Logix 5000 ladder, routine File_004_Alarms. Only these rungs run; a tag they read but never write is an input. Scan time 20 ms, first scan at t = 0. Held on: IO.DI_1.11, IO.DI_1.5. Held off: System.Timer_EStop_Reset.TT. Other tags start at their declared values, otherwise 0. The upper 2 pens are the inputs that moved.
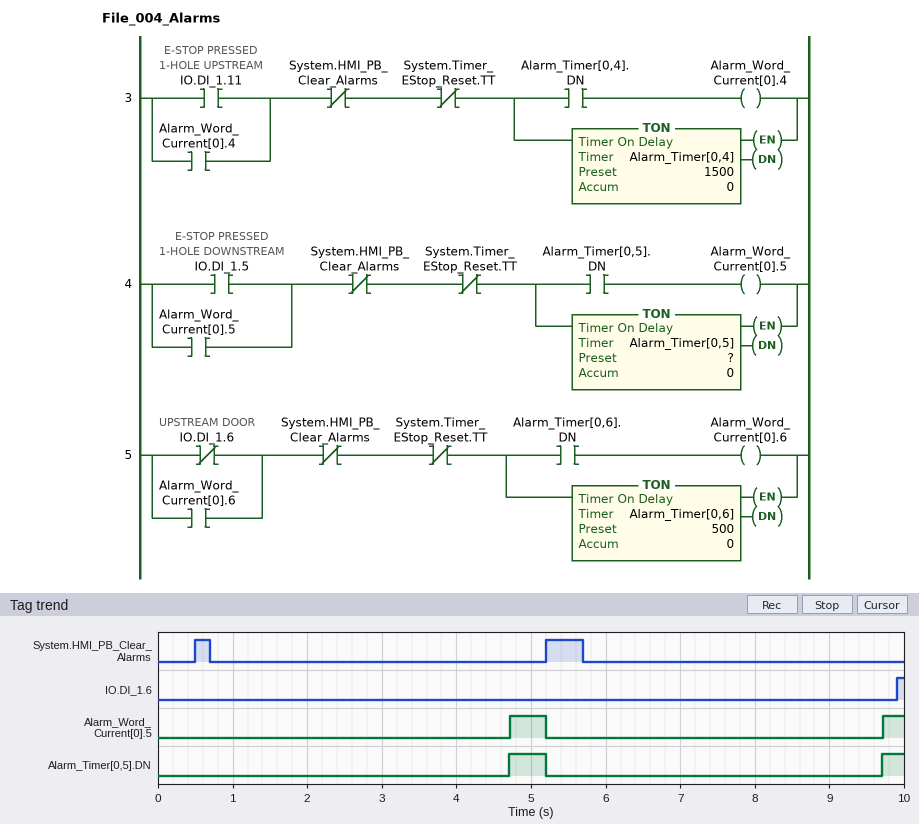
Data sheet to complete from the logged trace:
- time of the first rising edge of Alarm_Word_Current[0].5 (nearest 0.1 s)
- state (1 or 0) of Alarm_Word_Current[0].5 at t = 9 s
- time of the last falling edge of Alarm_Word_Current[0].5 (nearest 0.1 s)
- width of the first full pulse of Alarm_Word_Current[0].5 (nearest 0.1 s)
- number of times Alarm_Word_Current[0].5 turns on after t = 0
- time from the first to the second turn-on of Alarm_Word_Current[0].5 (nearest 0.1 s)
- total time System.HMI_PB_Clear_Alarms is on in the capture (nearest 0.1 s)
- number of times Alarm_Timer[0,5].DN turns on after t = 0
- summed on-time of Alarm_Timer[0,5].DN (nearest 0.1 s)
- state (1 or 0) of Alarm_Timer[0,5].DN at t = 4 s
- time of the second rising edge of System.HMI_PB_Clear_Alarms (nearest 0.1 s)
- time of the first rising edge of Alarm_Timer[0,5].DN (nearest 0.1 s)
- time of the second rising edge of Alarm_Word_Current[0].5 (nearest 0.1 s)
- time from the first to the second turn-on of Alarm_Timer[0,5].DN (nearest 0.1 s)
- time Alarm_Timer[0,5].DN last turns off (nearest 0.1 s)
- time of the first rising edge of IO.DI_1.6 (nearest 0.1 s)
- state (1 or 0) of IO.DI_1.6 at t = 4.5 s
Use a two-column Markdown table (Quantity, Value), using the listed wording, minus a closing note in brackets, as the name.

| Quantity | Value |
|---|---|
| time of the first rising edge of Alarm_Word_Current[0].5 | 4.7 s |
| state (1 or 0) of Alarm_Word_Current[0].5 at t = 9 s | 0 |
| time of the last falling edge of Alarm_Word_Current[0].5 | 5.2 s |
| width of the first full pulse of Alarm_Word_Current[0].5 | 0.5 s |
| number of times Alarm_Word_Current[0].5 turns on after t = 0 | 2 |
| time from the first to the second turn-on of Alarm_Word_Current[0].5 | 5.0 s |
| total time System.HMI_PB_Clear_Alarms is on in the capture | 0.7 s |
| number of times Alarm_Timer[0,5].DN turns on after t = 0 | 2 |
| summed on-time of Alarm_Timer[0,5].DN | 0.8 s |
| state (1 or 0) of Alarm_Timer[0,5].DN at t = 4 s | 0 |
| time of the second rising edge of System.HMI_PB_Clear_Alarms | 5.2 s |
| time of the first rising edge of Alarm_Timer[0,5].DN | 4.7 s |
| time of the second rising edge of Alarm_Word_Current[0].5 | 9.7 s |
| time from the first to the second turn-on of Alarm_Timer[0,5].DN | 5.0 s |
| time Alarm_Timer[0,5].DN last turns off | 5.2 s |
| time of the first rising edge of IO.DI_1.6 | 9.9 s |
| state (1 or 0) of IO.DI_1.6 at t = 4.5 s | 0 |
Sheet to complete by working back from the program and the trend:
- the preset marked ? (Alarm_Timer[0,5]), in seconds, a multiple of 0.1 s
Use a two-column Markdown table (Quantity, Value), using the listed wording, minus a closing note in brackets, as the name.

| Quantity | Value |
|---|---|
| the preset marked ? (Alarm_Timer[0,5]), in seconds, a multiple of 0.1 s | 4.0 s |
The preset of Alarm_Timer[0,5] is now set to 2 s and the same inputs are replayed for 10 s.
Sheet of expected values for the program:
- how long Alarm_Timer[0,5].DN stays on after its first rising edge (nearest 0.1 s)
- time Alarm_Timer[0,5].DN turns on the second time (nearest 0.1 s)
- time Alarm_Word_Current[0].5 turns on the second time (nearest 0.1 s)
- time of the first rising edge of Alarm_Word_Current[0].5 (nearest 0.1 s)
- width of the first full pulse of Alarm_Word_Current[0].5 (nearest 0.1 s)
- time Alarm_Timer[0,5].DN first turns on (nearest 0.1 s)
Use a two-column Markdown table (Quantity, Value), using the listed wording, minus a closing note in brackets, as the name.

| Quantity | Value |
|---|---|
| how long Alarm_Timer[0,5].DN stays on after its first rising edge | 2.5 s |
| time Alarm_Timer[0,5].DN turns on the second time | 7.7 s |
| time Alarm_Word_Current[0].5 turns on the second time | 7.7 s |
| time of the first rising edge of Alarm_Word_Current[0].5 | 2.7 s |
| width of the first full pulse of Alarm_Word_Current[0].5 | 2.5 s |
| time Alarm_Timer[0,5].DN first turns on | 2.7 s |
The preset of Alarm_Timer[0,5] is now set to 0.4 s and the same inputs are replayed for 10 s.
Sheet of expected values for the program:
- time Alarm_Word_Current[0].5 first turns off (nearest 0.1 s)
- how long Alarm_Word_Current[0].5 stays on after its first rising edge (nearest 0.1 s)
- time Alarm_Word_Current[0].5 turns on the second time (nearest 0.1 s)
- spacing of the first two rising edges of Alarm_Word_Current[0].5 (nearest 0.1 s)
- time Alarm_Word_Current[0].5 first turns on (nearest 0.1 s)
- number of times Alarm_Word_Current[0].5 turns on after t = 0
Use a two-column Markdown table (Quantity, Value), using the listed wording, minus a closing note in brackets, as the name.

| Quantity | Value |
|---|---|
| time Alarm_Word_Current[0].5 first turns off | 0.5 s |
| how long Alarm_Word_Current[0].5 stays on after its first rising edge | 0.1 s |
| time Alarm_Word_Current[0].5 turns on the second time | 1.1 s |
| spacing of the first two rising edges of Alarm_Word_Current[0].5 | 0.7 s |
| time Alarm_Word_Current[0].5 first turns on | 0.4 s |
| number of times Alarm_Word_Current[0].5 turns on after t = 0 | 3 |
